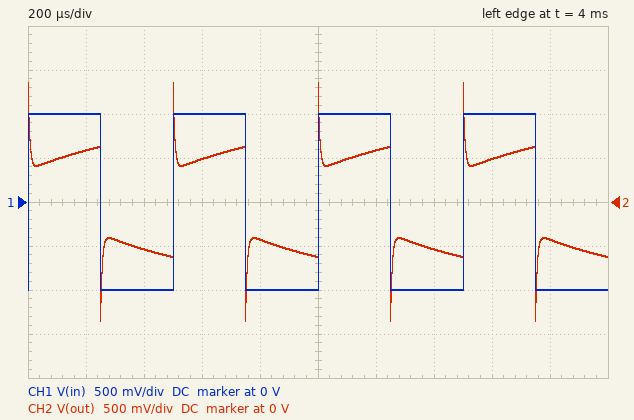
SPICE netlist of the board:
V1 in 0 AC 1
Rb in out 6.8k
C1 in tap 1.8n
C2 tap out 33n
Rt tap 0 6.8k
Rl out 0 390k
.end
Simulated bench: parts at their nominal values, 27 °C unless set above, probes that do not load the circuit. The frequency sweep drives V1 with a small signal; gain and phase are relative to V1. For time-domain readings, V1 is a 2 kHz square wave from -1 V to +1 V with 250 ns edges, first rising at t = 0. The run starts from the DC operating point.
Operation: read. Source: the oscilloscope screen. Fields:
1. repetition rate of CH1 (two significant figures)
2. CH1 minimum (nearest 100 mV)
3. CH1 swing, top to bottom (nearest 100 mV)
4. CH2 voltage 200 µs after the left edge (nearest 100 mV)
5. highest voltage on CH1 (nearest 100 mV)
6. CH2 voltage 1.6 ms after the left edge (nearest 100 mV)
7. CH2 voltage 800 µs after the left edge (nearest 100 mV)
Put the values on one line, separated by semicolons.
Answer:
2.0 kHz; -1.0 V; 2.0 V; 600 mV; 1.0 V; 500 mV; -400 mV
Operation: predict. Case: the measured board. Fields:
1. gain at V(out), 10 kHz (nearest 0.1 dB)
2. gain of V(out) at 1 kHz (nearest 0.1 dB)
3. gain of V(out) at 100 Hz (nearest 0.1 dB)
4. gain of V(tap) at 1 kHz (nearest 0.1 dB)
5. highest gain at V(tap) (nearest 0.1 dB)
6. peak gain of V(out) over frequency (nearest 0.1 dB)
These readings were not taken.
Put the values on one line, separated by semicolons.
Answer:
-4.8 dB; -4.9 dB; -0.4 dB; -6.2 dB; 0 dB; 0 dB
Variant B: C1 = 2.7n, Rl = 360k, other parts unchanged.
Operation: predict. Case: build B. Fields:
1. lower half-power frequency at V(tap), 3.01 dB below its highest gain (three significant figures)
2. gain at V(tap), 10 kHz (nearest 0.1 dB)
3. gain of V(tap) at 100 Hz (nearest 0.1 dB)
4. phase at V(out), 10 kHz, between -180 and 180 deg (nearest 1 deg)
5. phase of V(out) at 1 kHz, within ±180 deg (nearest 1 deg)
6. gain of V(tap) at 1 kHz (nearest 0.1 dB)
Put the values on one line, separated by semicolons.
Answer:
12.0 kHz; -3.5 dB; -16.8 dB; 18 deg; -13 deg; -6.1 dB
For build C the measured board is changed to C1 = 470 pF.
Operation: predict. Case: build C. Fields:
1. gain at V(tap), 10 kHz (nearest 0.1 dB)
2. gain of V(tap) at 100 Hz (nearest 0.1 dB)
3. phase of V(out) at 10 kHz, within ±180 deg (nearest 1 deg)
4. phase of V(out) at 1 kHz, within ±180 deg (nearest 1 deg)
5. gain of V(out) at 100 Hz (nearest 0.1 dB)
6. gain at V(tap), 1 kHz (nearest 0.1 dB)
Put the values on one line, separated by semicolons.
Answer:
-5.9 dB; -17.4 dB; 4 deg; -15 deg; -0.4 dB; -6.5 dB
